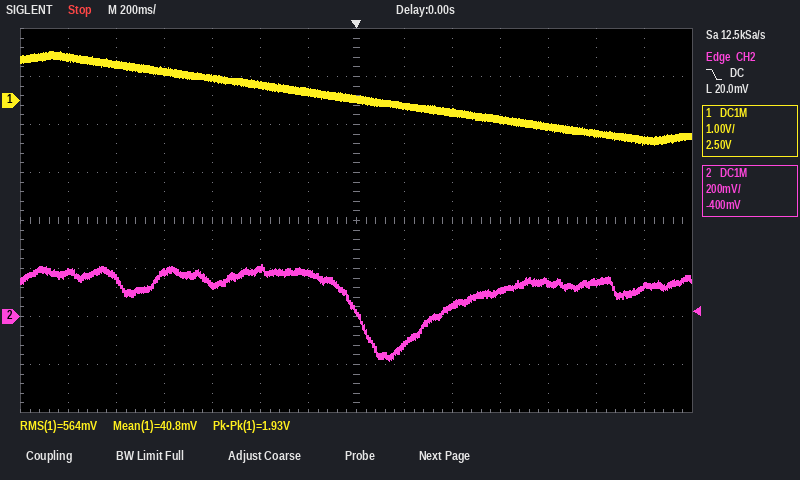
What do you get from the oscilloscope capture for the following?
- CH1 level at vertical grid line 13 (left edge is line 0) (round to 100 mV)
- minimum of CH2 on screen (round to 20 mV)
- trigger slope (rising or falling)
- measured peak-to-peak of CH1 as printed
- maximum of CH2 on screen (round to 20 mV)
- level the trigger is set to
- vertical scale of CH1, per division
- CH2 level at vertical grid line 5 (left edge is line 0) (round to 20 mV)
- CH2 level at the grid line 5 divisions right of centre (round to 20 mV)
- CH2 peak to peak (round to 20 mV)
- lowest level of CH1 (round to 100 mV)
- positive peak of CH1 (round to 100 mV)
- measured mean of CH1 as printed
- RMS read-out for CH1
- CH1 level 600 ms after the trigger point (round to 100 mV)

-800 mV
-180 mV
falling
1.93 V
220 mV
20.0 mV
1 V
200 mV
140 mV
400 mV
-900 mV
1.0 V
40.8 mV
564 mV
-400 mV
